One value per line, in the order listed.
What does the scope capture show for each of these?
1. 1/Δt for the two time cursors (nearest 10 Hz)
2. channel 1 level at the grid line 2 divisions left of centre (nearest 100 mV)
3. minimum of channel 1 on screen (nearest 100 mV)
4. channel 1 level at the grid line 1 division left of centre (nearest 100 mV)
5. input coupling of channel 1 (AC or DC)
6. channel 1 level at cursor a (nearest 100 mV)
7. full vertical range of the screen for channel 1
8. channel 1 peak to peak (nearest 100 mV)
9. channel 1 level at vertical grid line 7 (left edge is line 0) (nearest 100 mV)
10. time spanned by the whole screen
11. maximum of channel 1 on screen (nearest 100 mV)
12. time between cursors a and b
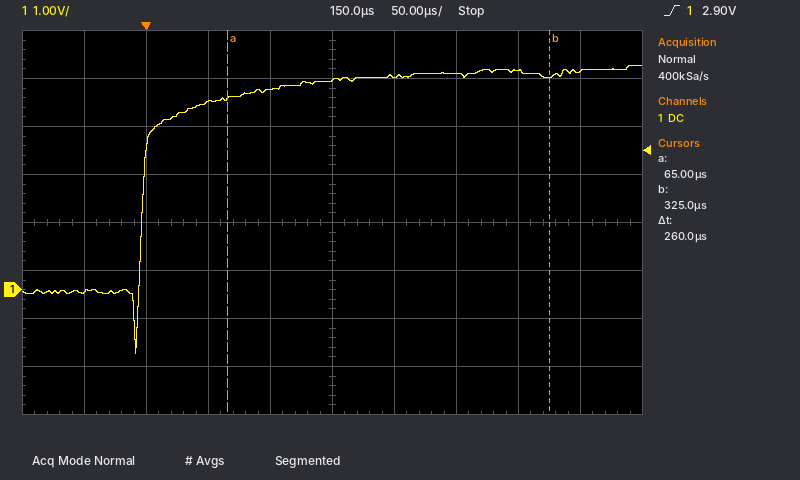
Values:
3.85 kHz
3.9 V
-1.3 V
4.2 V
DC
4.0 V
8 V
6.0 V
4.5 V
500 µs
4.7 V
260 µs
